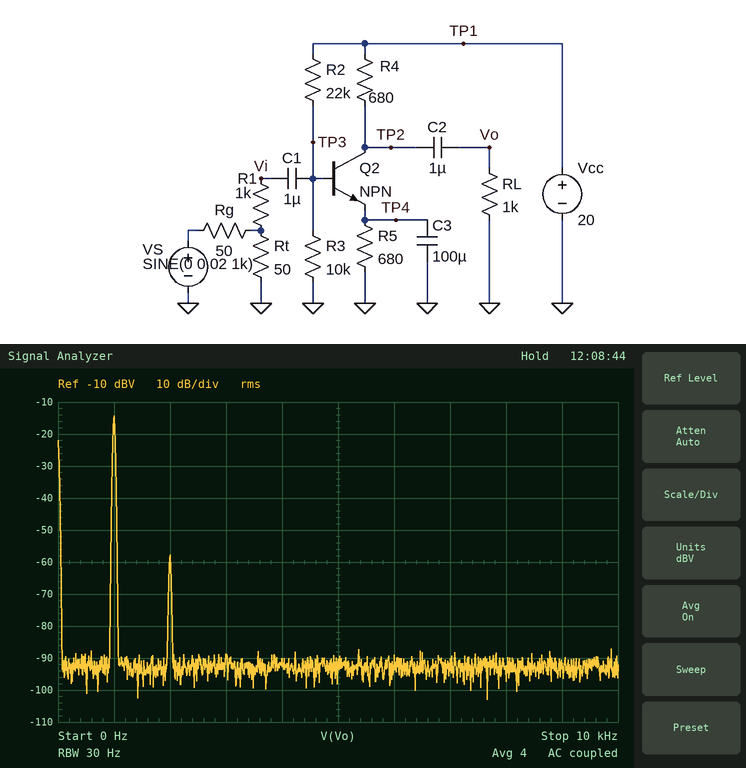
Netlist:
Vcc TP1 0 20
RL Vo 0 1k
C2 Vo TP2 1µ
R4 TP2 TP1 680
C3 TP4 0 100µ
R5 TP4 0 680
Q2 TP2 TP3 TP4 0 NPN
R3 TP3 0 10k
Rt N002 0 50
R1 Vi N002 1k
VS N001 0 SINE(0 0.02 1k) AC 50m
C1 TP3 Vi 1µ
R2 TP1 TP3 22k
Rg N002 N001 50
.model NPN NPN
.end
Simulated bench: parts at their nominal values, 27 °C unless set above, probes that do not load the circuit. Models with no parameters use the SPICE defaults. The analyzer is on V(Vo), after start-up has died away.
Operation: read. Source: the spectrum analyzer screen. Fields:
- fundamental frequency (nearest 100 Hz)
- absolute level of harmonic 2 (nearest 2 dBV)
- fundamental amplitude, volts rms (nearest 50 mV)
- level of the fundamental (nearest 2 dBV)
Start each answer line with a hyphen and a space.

- 1.0 kHz
- -58 dBV
- 200 mV
- -14 dBV
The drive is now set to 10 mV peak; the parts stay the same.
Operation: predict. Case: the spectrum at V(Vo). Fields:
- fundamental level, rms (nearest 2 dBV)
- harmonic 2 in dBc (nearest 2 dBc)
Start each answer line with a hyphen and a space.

- -20 dBV
- -50 dBc
